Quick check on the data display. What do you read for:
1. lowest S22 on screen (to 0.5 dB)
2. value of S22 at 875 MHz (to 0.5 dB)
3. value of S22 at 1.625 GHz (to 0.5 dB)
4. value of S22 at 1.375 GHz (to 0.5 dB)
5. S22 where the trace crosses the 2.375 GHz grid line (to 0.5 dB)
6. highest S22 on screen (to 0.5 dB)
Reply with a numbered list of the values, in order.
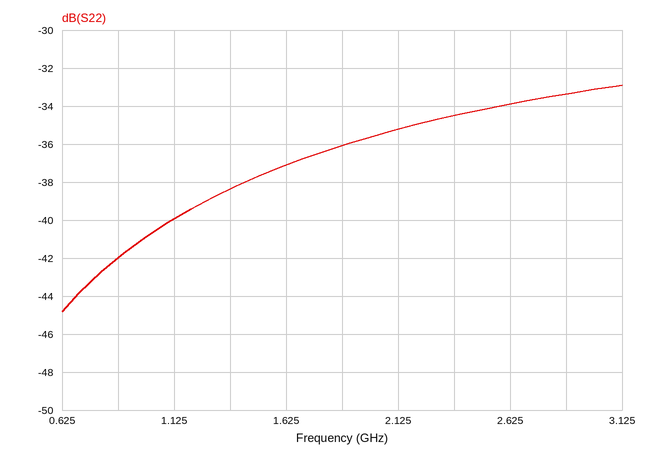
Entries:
1. -45.0 dB
2. -42.0 dB
3. -37.0 dB
4. -38.5 dB
5. -34.5 dB
6. -33.0 dB
